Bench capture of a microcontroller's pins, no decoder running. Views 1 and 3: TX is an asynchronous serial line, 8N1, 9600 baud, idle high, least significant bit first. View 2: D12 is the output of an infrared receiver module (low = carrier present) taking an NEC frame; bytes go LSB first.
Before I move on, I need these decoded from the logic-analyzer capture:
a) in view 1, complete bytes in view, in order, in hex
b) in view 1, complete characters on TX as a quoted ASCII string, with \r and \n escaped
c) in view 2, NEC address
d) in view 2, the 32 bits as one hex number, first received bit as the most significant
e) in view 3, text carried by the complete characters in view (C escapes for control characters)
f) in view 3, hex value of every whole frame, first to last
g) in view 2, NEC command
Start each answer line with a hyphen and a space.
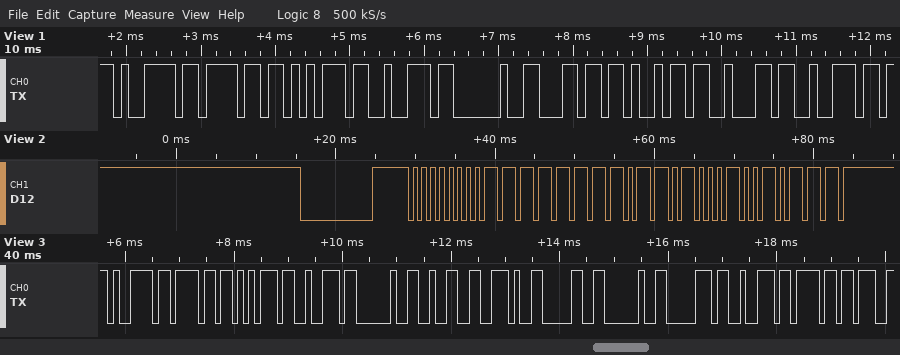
- 0x79 0x6F 0x75 0x72 0x20 0x6C 0x69 0x62 0x72
- "your libr"
- 0x00
- 0x00FF6897
- "your 2.0 pro"
- 79 6F 75 72 20 32 2E 30 20 70 72 6F
- 0x16
